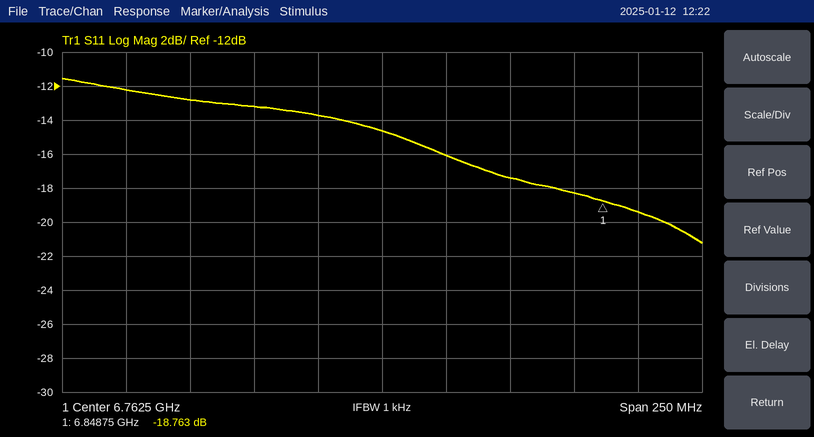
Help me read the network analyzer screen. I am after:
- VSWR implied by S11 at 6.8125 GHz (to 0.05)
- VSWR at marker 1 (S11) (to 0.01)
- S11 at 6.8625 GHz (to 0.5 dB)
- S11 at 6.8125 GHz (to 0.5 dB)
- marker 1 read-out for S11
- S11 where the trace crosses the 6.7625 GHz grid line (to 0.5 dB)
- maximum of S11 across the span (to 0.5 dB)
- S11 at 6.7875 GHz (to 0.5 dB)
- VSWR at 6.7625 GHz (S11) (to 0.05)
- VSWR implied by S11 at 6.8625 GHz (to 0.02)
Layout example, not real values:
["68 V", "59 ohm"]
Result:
["1.30", "1.26", "-19.5 dB", "-17.5 dB", "-18.763 dB", "-14.5 dB", "-11.5 dB", "-16.0 dB", "1.45", "1.24"]
